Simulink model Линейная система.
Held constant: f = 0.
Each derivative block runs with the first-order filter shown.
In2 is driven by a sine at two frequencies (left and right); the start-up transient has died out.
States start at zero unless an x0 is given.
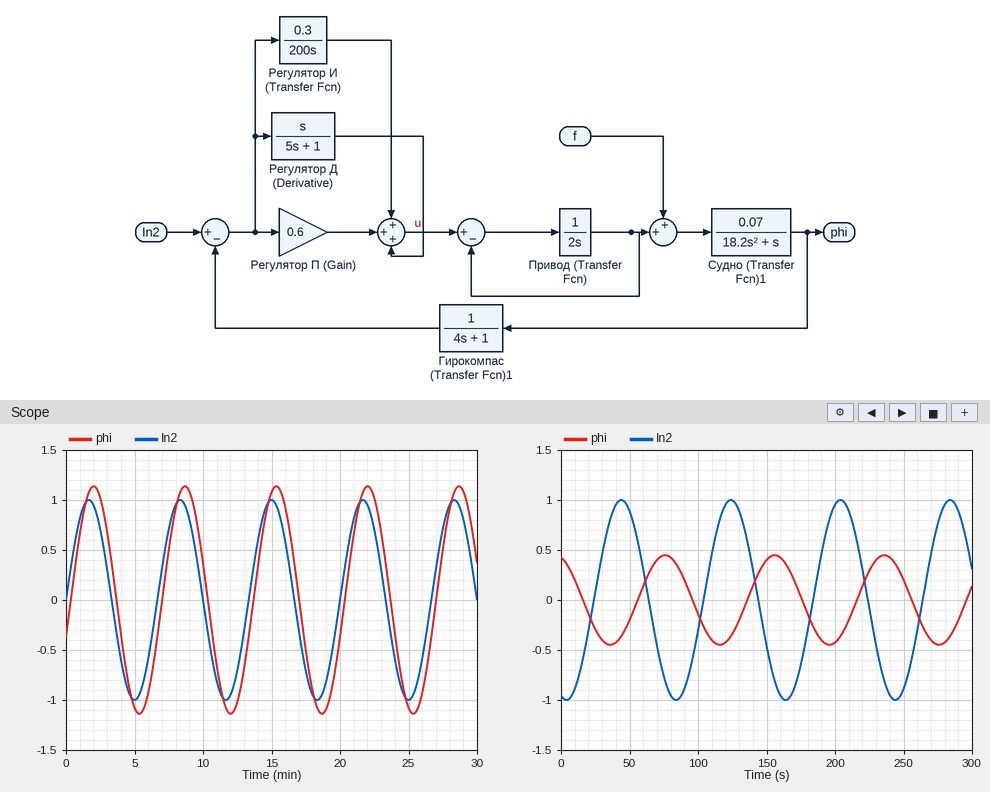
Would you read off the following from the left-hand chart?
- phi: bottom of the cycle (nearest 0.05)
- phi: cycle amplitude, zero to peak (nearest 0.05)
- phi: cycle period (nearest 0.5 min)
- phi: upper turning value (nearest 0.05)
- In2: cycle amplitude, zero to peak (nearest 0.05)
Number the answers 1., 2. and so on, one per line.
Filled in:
1. -1.15
2. 1.15
3. 6.5 min
4. 1.15
5. 1.00
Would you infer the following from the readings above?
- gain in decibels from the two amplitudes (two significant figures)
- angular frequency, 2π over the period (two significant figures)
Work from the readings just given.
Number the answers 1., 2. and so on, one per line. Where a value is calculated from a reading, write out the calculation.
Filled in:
1. 20 log10(1.15 / 1) = 1.2 dB
2. 2π / 6.5 = 0.97 rad/min
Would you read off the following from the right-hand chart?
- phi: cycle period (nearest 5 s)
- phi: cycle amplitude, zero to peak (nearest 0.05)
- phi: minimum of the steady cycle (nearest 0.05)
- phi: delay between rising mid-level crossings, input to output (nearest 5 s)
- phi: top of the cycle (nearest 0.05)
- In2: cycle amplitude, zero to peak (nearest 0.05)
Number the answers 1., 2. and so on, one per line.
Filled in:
1. 80 s
2. 0.45
3. -0.45
4. 30 s
5. 0.45
6. 1.00
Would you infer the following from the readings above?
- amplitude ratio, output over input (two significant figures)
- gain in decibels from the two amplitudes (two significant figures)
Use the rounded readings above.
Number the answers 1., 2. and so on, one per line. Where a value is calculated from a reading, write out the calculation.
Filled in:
1. 0.45 / 1 = 0.45
2. 20 log10(0.45 / 1) = -6.9 dB
